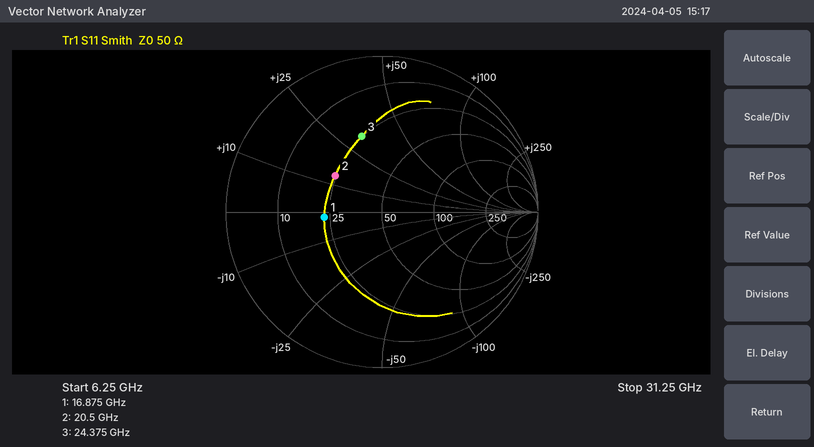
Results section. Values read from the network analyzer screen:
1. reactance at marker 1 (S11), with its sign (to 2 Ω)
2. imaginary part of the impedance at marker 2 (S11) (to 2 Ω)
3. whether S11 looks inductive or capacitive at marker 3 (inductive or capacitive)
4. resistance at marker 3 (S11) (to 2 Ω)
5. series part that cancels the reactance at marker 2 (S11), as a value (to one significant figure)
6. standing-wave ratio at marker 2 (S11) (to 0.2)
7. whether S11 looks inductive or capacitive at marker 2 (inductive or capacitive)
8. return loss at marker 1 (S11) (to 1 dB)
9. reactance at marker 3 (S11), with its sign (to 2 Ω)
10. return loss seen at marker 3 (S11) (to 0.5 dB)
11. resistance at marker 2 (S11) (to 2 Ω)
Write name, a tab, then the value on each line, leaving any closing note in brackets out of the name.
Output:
reactance at marker 1 (S11), with its sign	-2 Ω
imaginary part of the impedance at marker 2 (S11)	+14 Ω
whether S11 looks inductive or capacitive at marker 3	inductive
resistance at marker 3 (S11)	24 Ω
series part that cancels the reactance at marker 2 (S11), as a value	600 fF
standing-wave ratio at marker 2 (S11)	2.2
whether S11 looks inductive or capacitive at marker 2	inductive
return loss at marker 1 (S11)	9 dB
reactance at marker 3 (S11), with its sign	+32 Ω
return loss seen at marker 3 (S11)	6.0 dB
resistance at marker 2 (S11)	24 Ω
